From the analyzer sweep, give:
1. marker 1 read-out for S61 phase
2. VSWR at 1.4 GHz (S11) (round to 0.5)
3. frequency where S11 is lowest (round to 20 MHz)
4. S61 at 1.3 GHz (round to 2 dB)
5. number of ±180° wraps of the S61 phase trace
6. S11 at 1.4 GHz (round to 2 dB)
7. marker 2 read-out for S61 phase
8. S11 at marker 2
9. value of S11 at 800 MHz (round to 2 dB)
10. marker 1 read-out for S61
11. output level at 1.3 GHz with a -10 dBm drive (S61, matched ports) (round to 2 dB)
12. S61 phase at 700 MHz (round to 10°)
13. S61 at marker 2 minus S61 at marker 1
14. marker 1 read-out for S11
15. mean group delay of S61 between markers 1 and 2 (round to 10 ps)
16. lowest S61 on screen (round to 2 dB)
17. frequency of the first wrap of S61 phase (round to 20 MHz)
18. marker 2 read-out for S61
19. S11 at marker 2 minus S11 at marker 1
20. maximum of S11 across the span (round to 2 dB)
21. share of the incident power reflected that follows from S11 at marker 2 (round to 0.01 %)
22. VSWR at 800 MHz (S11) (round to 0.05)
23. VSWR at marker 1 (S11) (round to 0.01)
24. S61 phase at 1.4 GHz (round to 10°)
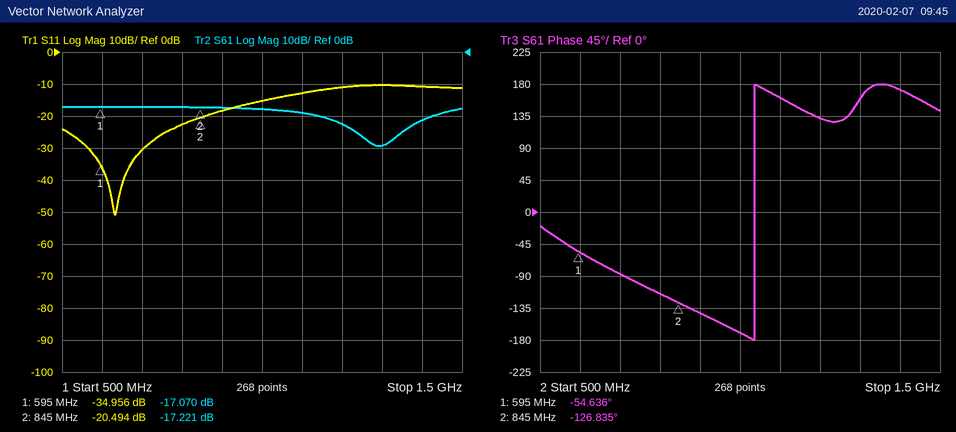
-54.636°
2.0
640 MHz
-30 dB
1
-10 dB
-126.835°
-20.494 dB
-22 dB
-17.070 dB
-40 dBm
-90°
-0.151 dB
-34.956 dB
800 ps
-30 dB
1.04 GHz
-17.221 dB
14.462 dB
-10 dB
0.89 %
1.15
1.04
170°
